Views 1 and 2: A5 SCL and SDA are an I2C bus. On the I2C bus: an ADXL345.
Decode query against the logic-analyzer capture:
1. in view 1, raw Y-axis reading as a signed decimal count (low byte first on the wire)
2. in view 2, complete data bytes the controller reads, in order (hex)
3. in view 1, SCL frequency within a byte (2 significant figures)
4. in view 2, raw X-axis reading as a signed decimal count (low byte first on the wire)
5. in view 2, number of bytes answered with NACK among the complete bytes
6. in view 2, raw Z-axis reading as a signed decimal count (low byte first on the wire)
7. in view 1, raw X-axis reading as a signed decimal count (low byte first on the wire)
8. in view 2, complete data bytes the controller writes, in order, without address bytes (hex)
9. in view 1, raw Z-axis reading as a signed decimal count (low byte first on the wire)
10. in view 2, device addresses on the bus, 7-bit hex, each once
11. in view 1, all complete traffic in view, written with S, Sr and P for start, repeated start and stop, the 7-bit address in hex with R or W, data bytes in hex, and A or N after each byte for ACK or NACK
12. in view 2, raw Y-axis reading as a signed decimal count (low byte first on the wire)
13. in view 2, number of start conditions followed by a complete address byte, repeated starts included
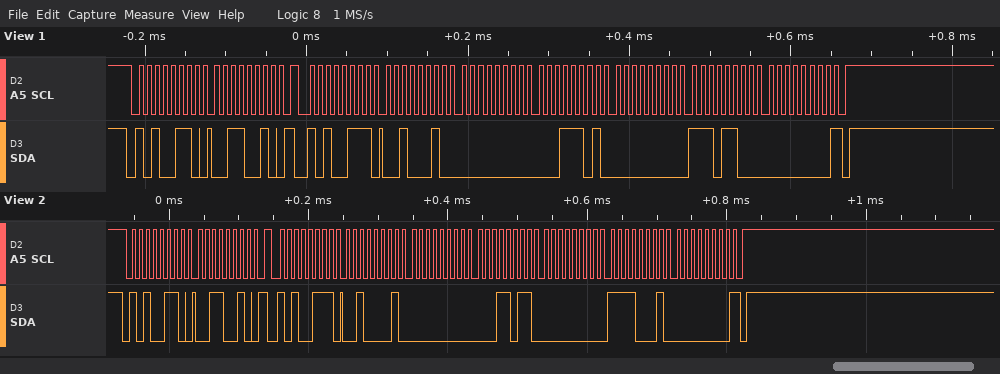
29
21 00 1B 00 F1 00
100 kHz
33
1
241
34
32
236
0x53
S 53W A 32 A Sr 53R A 22 A 00 A 1D A 00 A EC A 00 N P
27
2
